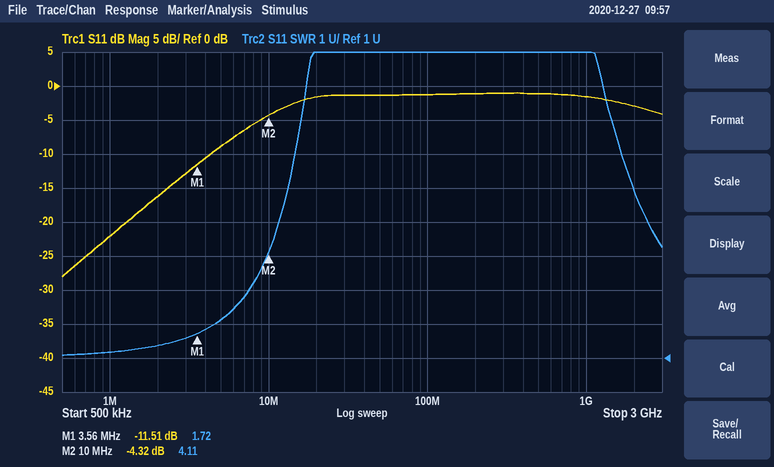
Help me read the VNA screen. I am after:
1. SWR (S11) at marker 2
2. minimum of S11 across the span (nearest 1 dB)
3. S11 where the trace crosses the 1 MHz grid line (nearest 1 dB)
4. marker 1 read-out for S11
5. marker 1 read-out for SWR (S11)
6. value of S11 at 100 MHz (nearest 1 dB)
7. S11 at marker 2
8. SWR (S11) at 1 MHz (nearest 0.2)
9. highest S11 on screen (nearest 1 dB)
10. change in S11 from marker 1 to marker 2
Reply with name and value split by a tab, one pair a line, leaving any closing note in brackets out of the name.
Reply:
SWR (S11) at marker 2	4.11
minimum of S11 across the span	-28 dB
S11 where the trace crosses the 1 MHz grid line	-22 dB
marker 1 read-out for S11	-11.51 dB
marker 1 read-out for SWR	1.72
value of S11 at 100 MHz	-1 dB
S11 at marker 2	-4.32 dB
SWR (S11) at 1 MHz	1.2
highest S11 on screen	-1 dB
change in S11 from marker 1 to marker 2	7.19 dB
